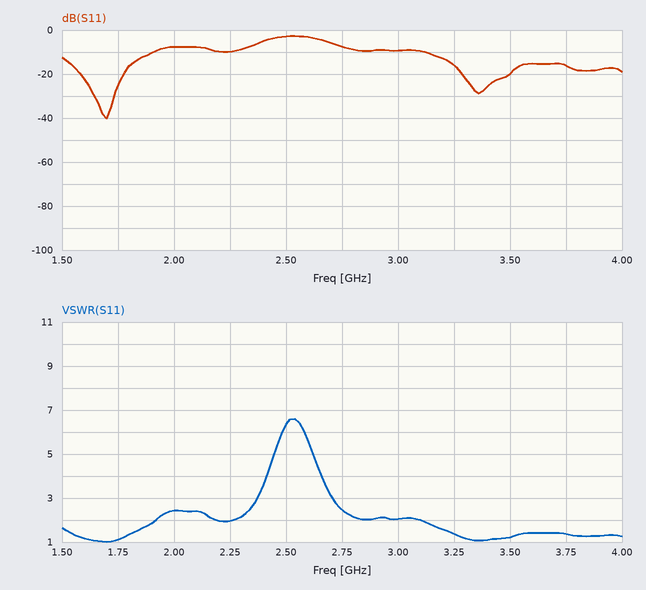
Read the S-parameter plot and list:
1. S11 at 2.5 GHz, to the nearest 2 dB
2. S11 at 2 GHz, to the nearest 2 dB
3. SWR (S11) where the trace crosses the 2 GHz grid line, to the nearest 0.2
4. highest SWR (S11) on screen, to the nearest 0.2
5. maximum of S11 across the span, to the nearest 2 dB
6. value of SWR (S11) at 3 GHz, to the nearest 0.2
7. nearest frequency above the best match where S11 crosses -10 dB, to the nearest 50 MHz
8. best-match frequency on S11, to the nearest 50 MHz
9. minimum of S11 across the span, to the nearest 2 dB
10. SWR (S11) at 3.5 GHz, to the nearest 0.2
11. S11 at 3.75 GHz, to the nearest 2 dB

-2 dB
-8 dB
2.4
6.6
-2 dB
2.0
1.90 GHz
1.70 GHz
-40 dB
1.2
-16 dB
